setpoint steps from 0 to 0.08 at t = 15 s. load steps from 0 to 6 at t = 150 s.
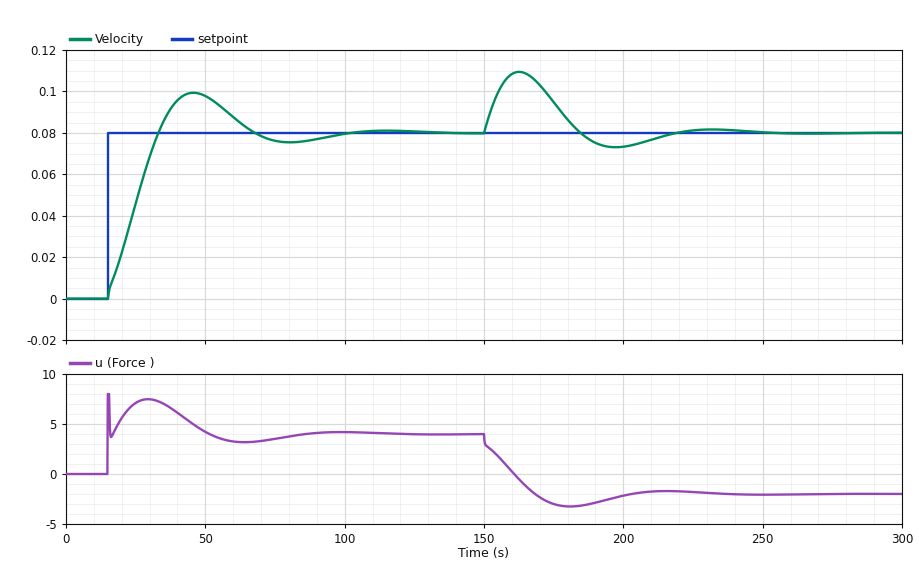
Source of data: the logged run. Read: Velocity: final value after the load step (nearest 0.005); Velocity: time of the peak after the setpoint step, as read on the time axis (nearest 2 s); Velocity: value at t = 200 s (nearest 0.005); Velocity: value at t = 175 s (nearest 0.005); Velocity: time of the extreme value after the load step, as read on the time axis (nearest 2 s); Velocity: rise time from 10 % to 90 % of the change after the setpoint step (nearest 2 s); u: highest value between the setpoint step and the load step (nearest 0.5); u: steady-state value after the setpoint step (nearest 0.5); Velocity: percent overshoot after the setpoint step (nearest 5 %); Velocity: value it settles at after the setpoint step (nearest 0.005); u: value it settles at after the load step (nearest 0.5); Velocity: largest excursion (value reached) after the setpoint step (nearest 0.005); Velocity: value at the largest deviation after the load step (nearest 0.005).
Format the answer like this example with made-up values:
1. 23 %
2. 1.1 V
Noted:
1. 0.080
2. 46 s
3. 0.075
4. 0.095
5. 162 s
6. 14 s
7. 8.0
8. 4.0
9. 25 %
10. 0.080
11. -2.0
12. 0.100
13. 0.110
